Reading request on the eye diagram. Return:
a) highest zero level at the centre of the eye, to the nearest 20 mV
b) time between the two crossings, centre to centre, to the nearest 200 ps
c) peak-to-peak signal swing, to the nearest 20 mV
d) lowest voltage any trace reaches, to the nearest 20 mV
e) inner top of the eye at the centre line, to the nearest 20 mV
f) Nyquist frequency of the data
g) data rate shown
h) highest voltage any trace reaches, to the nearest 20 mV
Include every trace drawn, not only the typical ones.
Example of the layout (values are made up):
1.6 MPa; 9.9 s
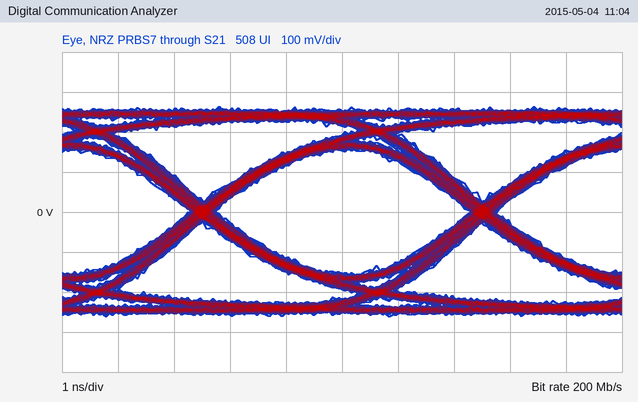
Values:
-160 mV; 5.0 ns; 520 mV; -260 mV; 160 mV; 100 MHz; 200 Mb/s; 260 mV
